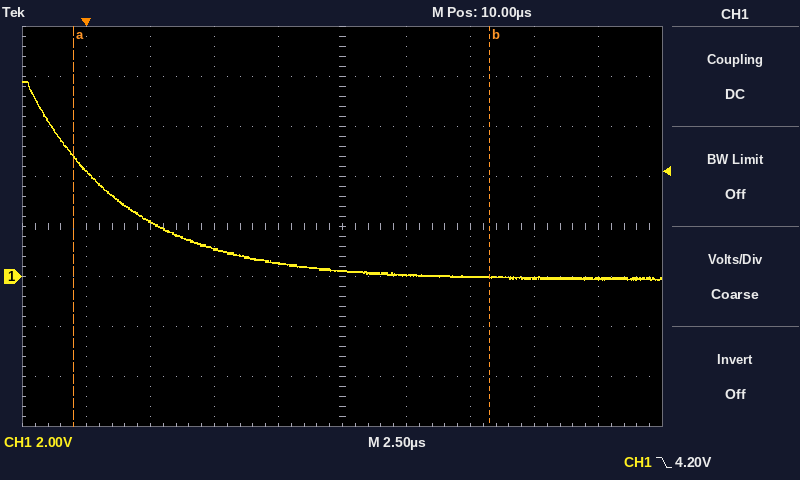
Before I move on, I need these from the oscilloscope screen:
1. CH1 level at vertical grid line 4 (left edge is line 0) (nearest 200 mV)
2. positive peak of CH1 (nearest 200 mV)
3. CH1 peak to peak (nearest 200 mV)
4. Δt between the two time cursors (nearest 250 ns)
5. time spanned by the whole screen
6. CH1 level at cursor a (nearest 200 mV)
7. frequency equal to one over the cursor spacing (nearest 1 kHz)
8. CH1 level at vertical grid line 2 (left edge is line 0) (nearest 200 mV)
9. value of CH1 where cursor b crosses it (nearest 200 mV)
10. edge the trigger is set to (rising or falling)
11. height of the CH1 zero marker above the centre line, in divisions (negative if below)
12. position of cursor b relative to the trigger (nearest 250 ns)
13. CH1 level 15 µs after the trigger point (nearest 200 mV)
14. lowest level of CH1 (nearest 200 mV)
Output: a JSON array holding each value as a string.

["600 mV", "7.8 V", "8.0 V", "16.25 µs", "25 µs", "4.8 V", "62 kHz", "2.2 V", "0.0 V", "falling", "-1.0 div", "+15.75 µs", "0.0 V", "-200 mV"]
